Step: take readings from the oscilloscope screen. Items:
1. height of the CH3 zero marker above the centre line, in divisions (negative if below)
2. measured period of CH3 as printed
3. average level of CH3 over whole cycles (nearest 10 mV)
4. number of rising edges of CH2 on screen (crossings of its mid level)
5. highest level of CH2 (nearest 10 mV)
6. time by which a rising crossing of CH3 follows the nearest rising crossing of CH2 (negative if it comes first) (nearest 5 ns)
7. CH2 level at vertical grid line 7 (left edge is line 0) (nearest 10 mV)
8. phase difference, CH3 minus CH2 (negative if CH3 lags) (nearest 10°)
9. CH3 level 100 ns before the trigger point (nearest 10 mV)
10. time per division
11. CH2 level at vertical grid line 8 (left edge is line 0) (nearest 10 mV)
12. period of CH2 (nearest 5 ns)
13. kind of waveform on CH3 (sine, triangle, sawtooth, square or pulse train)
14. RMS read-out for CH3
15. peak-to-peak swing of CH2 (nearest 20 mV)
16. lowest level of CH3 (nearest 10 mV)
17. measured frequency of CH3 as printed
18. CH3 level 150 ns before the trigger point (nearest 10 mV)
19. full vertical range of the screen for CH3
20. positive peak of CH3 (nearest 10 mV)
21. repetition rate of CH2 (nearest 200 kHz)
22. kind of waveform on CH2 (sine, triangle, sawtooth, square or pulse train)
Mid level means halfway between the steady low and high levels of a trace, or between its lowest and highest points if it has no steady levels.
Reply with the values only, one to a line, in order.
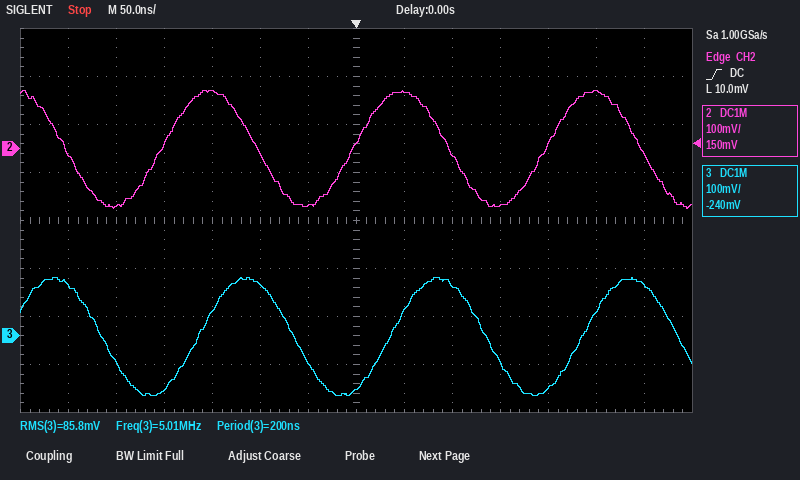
-2.4 div
200 ns
0 mV
3
120 mV
+40 ns
10 mV
-70°
110 mV
50 ns
120 mV
200 ns
sine
85.8 mV
240 mV
-120 mV
5.01 MHz
50 mV
800 mV
120 mV
5.0 MHz
sine
